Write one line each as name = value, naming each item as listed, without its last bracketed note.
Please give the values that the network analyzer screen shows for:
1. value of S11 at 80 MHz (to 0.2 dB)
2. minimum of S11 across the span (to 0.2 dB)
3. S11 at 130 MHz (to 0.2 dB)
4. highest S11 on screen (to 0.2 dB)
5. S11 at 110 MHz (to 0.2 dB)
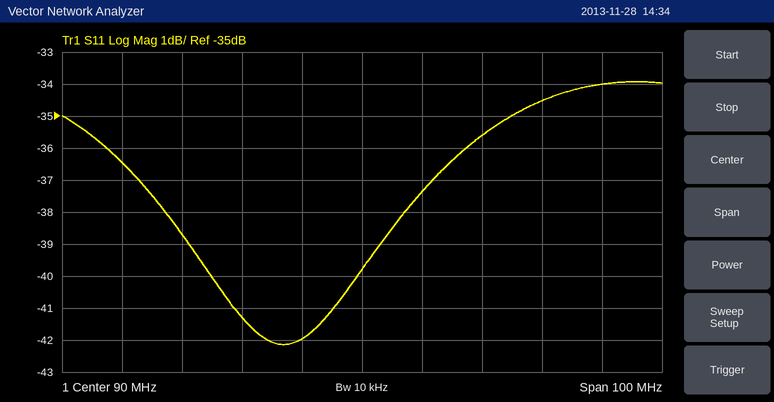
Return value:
value of S11 at 80 MHz = -42.0 dB
minimum of S11 across the span = -42.2 dB
S11 at 130 MHz = -34.0 dB
highest S11 on screen = -34.0 dB
S11 at 110 MHz = -35.6 dB
